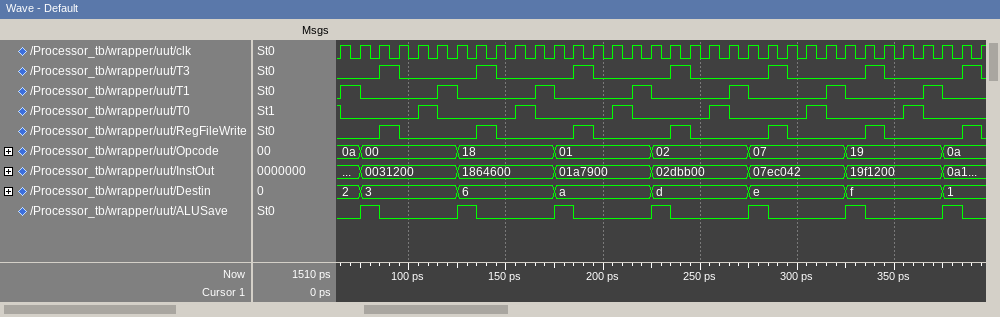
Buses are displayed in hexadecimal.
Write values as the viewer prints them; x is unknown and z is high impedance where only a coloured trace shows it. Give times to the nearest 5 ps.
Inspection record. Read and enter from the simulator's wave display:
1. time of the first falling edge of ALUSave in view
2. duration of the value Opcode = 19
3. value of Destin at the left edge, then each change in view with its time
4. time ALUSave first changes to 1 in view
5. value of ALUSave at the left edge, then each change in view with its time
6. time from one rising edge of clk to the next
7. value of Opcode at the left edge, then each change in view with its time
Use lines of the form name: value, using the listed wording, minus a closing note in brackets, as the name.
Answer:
time of the first falling edge of ALUSave in view: 85 ps
duration of the value Opcode = 19: 50 ps
value of Destin at the left edge, then each change in view with its time: 2, 3 at 75 ps, 6 at 125 ps, a at 175 ps, d at 225 ps, e at 275 ps, f at 325 ps, 1 at 375 ps
time ALUSave first changes to 1 in view: 75 ps
value of ALUSave at the left edge, then each change in view with its time: 0, 1 at 75 ps, 0 at 85 ps, 1 at 125 ps, 0 at 135 ps, 1 at 175 ps, 0 at 185 ps, 1 at 225 ps, 0 at 235 ps, 1 at 275 ps, 0 at 285 ps, 1 at 325 ps, 0 at 335 ps, 1 at 375 ps, 0 at 385 ps
time from one rising edge of clk to the next: 10 ps
value of Opcode at the left edge, then each change in view with its time: 0a, 00 at 75 ps, 18 at 125 ps, 01 at 175 ps, 02 at 225 ps, 07 at 275 ps, 19 at 325 ps, 0a at 375 ps
